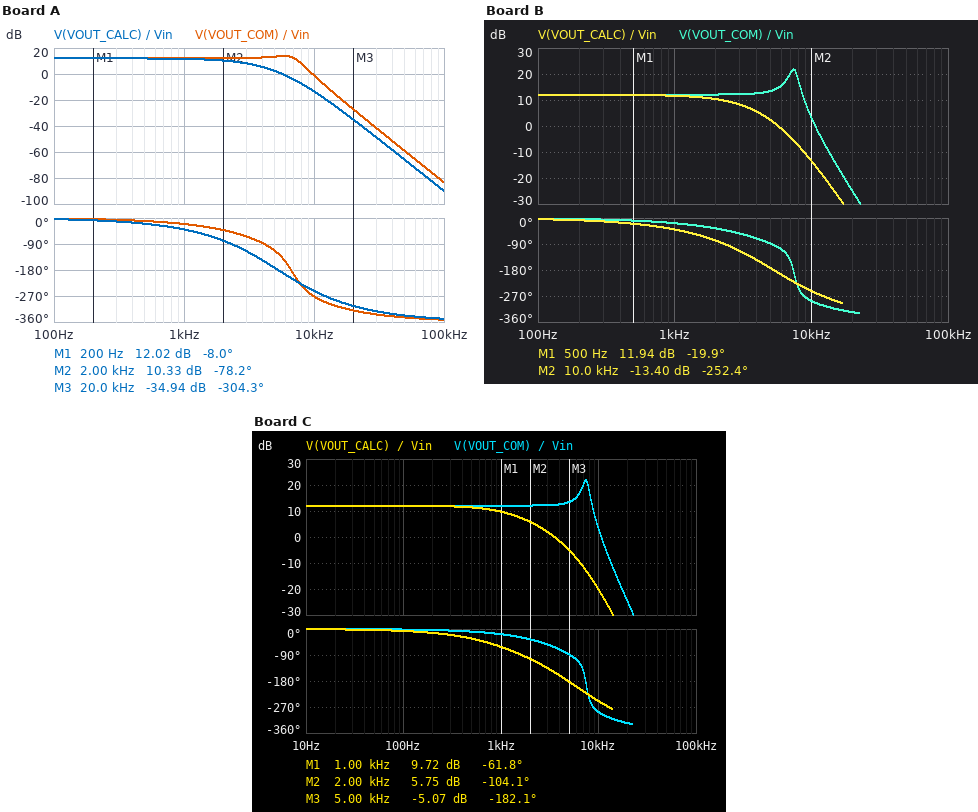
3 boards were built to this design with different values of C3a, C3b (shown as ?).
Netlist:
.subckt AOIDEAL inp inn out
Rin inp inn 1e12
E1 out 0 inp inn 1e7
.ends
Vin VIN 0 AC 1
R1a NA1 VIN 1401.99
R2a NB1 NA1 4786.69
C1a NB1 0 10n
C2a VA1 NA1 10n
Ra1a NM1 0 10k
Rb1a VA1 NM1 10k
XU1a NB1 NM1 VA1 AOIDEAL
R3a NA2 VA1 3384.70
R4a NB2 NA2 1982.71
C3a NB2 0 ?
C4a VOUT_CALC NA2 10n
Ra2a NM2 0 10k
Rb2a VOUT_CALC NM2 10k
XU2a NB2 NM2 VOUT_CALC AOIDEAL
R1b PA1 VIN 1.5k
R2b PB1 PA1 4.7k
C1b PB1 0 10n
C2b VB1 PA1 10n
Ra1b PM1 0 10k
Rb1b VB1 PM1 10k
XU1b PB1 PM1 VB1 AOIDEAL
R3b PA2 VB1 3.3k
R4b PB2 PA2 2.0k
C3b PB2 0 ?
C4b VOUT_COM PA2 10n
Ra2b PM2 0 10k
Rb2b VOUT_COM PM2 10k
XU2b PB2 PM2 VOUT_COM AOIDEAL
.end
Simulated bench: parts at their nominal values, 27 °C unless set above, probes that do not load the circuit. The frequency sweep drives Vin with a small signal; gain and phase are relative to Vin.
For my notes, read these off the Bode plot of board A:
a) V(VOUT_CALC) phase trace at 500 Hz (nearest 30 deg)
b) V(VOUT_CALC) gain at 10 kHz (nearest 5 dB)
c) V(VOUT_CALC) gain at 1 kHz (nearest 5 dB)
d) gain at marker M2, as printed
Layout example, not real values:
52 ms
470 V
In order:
-30 deg
-15 dB
10 dB
10.33 dB
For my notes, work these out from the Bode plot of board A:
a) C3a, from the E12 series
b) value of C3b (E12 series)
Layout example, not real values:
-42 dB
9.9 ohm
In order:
18 nF
8.2 nF
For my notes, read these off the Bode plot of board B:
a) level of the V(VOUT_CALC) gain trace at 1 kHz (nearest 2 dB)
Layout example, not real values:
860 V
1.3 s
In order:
12 dB
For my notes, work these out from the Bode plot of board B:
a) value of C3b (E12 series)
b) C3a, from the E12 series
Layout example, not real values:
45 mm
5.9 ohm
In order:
6.8 nF
18 nF
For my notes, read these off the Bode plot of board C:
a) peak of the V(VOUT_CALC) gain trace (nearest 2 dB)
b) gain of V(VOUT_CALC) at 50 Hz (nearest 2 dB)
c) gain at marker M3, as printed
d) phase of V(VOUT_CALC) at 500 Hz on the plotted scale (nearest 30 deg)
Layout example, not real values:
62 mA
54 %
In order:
12 dB
12 dB
-5.07 dB
-30 deg
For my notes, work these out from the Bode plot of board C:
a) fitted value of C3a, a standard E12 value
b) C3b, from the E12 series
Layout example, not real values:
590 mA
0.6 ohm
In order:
33 nF
6.8 nF
